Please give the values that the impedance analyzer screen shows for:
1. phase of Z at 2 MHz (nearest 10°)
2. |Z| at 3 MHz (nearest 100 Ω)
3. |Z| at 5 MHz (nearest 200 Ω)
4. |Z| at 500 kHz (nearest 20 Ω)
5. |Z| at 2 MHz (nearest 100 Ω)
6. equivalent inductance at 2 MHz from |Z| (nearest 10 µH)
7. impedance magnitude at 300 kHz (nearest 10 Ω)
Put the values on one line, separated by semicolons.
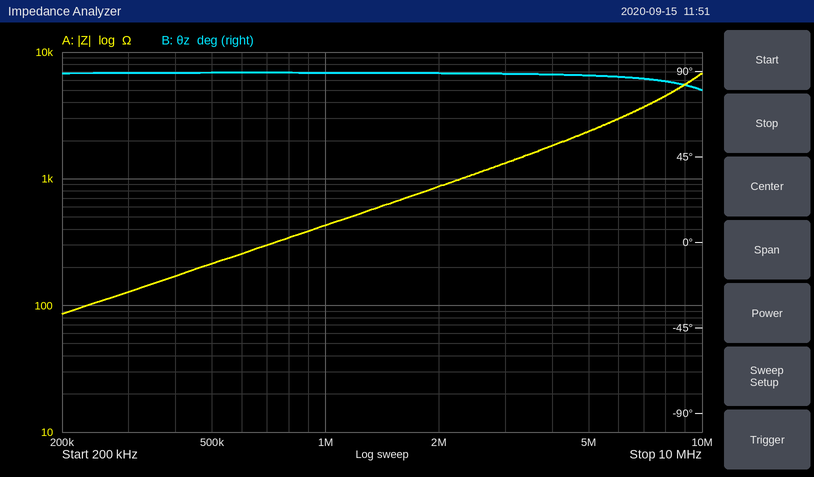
90°; 1.3 kΩ; 2.4 kΩ; 220 Ω; 900 Ω; 70 µH; 130 Ω
